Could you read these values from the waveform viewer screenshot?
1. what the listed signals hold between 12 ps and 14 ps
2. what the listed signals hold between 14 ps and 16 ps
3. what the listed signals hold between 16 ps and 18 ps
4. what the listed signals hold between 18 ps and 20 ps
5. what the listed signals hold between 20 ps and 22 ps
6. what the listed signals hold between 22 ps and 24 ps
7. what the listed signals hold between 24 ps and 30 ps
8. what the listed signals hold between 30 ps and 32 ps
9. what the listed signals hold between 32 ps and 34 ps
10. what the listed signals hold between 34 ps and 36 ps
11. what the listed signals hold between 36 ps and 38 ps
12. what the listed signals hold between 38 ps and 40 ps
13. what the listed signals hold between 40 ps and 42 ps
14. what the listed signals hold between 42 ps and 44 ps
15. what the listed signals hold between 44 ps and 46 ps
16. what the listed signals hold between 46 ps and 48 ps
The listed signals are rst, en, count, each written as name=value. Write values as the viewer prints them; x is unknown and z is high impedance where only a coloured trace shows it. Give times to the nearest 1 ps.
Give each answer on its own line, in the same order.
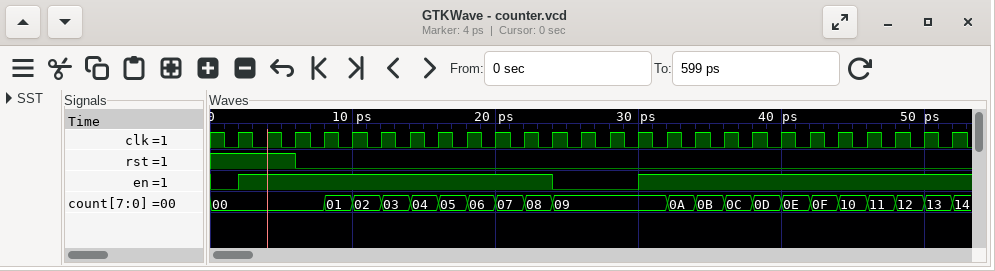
rst=0, en=1, count=03
rst=0, en=1, count=04
rst=0, en=1, count=05
rst=0, en=1, count=06
rst=0, en=1, count=07
rst=0, en=1, count=08
rst=0, en=0, count=09
rst=0, en=1, count=09
rst=0, en=1, count=0A
rst=0, en=1, count=0B
rst=0, en=1, count=0C
rst=0, en=1, count=0D
rst=0, en=1, count=0E
rst=0, en=1, count=0F
rst=0, en=1, count=10
rst=0, en=1, count=11
